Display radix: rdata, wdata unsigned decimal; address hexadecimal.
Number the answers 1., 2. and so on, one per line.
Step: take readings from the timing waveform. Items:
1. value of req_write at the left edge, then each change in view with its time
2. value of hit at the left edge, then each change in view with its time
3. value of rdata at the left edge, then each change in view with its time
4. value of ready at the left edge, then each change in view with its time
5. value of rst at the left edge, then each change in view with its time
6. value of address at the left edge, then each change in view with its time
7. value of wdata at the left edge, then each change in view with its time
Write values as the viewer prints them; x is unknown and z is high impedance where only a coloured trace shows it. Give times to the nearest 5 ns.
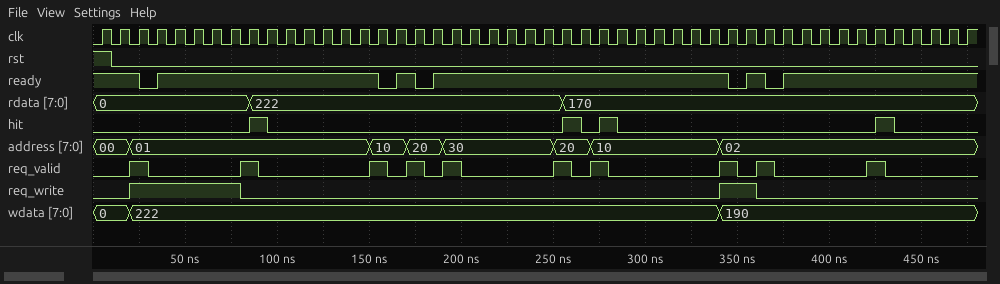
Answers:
1. 0, 1 at 20 ns, 0 at 80 ns, 1 at 340 ns, 0 at 360 ns
2. 0, 1 at 85 ns, 0 at 95 ns, 1 at 255 ns, 0 at 265 ns, 1 at 275 ns, 0 at 285 ns, 1 at 425 ns, 0 at 435 ns
3. 0, 222 at 85 ns, 170 at 255 ns
4. 1, 0 at 25 ns, 1 at 35 ns, 0 at 155 ns, 1 at 165 ns, 0 at 175 ns, 1 at 185 ns, 0 at 345 ns, 1 at 355 ns, 0 at 365 ns, 1 at 375 ns
5. 1, 0 at 10 ns
6. 00, 01 at 20 ns, 10 at 150 ns, 20 at 170 ns, 30 at 190 ns, 20 at 250 ns, 10 at 270 ns, 02 at 340 ns
7. 0, 222 at 20 ns, 190 at 340 ns
